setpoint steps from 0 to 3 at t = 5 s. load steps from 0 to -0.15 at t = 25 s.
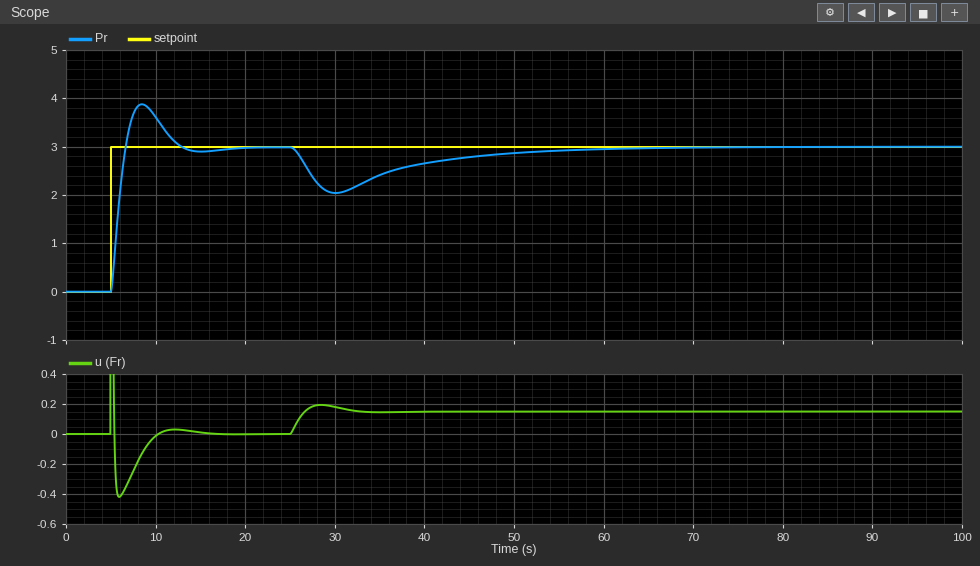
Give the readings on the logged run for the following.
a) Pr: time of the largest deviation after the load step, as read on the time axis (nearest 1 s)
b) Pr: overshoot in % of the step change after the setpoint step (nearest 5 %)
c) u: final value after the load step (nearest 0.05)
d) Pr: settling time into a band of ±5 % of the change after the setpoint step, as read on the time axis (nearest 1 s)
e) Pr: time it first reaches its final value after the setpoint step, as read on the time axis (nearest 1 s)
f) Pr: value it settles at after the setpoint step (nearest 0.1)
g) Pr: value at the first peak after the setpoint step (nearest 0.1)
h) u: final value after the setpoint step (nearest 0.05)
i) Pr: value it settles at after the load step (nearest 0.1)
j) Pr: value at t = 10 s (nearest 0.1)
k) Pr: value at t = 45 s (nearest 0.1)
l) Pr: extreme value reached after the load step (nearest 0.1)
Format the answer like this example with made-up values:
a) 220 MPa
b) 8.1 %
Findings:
a) 30 s
b) 30 %
c) 0.15
d) 12 s
e) 7 s
f) 3.0
g) 3.9
h) 0.00
i) 3.0
j) 3.6
k) 2.8
l) 2.0
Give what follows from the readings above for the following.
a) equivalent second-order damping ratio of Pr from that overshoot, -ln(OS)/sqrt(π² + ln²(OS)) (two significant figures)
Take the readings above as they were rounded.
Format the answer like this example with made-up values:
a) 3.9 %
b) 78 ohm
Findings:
a) 0.36
